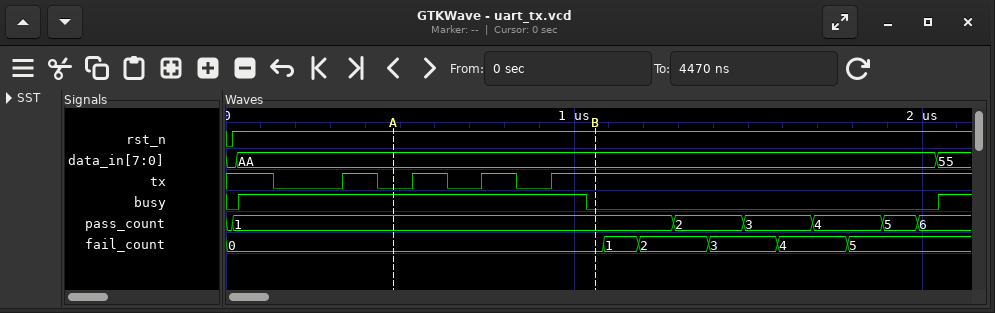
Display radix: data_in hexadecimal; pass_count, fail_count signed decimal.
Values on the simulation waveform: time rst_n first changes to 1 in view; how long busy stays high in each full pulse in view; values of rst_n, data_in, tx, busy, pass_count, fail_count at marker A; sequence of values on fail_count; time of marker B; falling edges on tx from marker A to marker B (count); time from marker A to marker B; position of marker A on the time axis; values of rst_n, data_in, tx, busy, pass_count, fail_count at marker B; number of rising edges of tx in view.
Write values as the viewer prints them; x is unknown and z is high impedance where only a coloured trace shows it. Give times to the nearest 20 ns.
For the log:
20 ns
1000 ns
rst_n=1, data_in=AA, tx=0, busy=1, pass_count=1, fail_count=0
0, 1, 2, 3, 4, 5
1060 ns
2
580 ns
480 ns
rst_n=1, data_in=AA, tx=1, busy=0, pass_count=1, fail_count=0
4
